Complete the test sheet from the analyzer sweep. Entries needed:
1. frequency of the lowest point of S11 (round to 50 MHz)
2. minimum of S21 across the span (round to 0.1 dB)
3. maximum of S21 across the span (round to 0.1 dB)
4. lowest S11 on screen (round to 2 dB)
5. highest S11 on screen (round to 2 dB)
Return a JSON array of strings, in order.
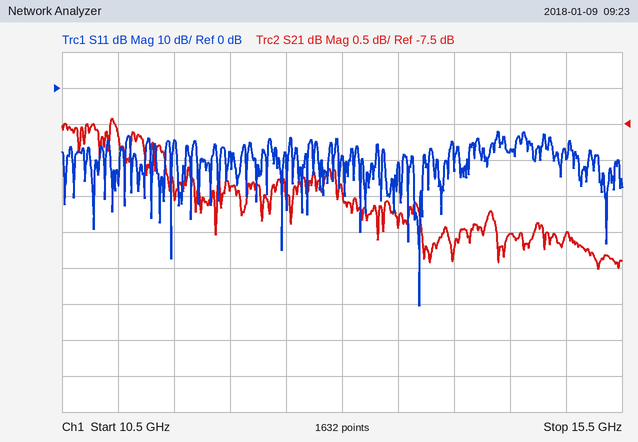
["13.70 GHz", "-9.5 dB", "-7.4 dB", "-60 dB", "-12 dB"]
